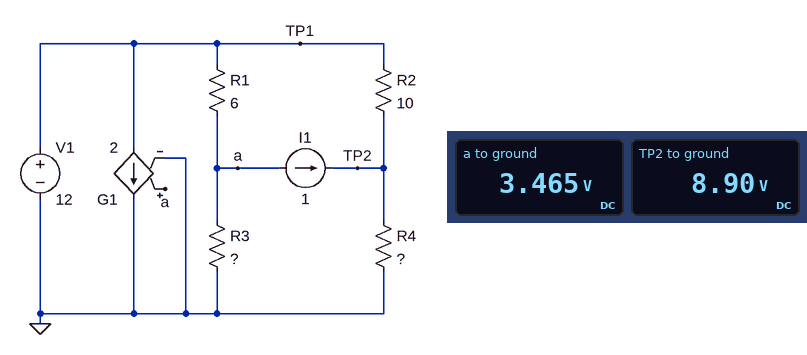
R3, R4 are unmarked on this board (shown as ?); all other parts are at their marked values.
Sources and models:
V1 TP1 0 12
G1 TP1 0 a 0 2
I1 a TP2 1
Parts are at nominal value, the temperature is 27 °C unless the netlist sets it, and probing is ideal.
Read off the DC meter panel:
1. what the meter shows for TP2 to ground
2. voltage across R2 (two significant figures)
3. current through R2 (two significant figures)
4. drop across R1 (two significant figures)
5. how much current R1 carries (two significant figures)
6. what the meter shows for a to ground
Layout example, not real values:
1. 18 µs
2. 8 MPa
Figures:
1. 8.90 V
2. 3.1 V
3. 310 mA
4. 8.5 V
5. 1.4 A
6. 3.465 V
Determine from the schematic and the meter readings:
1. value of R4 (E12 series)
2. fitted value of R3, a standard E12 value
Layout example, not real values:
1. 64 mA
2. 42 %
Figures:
1. 6.8 Ω
2. 8.2 Ω
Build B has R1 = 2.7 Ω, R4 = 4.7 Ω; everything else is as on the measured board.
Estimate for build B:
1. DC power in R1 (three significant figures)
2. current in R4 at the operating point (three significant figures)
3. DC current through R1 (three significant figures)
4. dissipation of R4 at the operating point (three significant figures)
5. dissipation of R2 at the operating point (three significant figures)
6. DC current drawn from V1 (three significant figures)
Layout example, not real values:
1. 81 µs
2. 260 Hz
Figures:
1. 9.27 W
2. 1.50 A
3. 1.85 A
4. 10.5 W
5. 2.47 W
6. 16.3 A
